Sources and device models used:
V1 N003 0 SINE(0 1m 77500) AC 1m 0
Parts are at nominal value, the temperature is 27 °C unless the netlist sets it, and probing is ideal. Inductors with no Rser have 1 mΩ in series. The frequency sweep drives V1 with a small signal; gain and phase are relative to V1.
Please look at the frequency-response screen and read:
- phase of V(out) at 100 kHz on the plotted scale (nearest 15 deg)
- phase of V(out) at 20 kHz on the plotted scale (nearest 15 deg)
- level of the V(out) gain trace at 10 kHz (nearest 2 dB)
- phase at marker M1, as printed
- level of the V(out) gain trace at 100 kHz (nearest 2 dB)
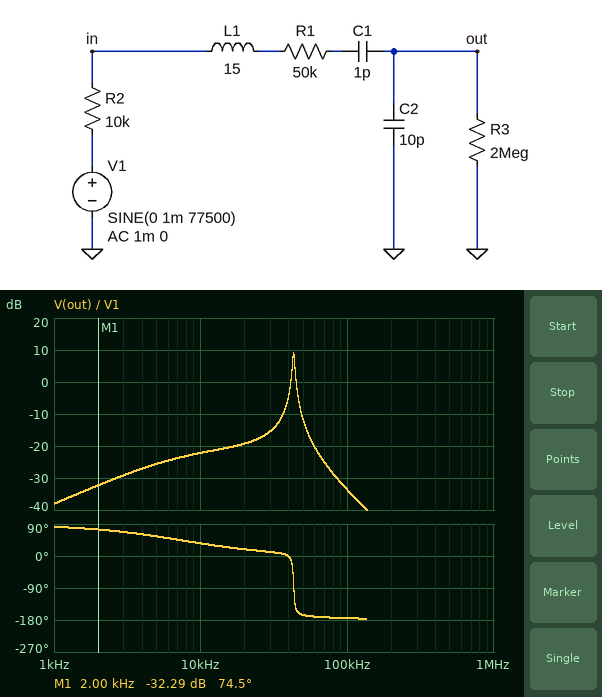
-180 deg
15 deg
-22 dB
74.5 deg
-34 dB
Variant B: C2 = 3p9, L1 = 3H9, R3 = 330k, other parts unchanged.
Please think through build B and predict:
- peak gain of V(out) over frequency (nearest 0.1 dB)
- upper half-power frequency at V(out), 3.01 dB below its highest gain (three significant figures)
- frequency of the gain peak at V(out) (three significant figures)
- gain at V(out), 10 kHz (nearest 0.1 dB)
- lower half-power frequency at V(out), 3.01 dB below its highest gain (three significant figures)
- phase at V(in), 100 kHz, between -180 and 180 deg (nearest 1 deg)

-0.4 dB
90.1 kHz
83.9 kHz
-33.6 dB
77.8 kHz
1 deg
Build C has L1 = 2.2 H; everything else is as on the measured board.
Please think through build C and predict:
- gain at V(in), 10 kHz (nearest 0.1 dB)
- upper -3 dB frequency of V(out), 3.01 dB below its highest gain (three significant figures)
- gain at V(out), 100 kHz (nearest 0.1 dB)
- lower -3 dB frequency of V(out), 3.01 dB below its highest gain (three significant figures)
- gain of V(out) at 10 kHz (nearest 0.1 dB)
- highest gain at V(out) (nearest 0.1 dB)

0 dB
115 kHz
-7.5 dB
110 kHz
-22.6 dB
6.1 dB
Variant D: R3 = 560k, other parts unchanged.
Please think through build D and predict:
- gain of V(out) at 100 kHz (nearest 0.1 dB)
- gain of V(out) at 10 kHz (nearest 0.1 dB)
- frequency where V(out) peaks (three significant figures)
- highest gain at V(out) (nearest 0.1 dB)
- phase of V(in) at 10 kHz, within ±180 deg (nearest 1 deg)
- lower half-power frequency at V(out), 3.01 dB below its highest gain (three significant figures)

-34.0 dB
-29.2 dB
42.5 kHz
2.5 dB
0 deg
41.2 kHz
